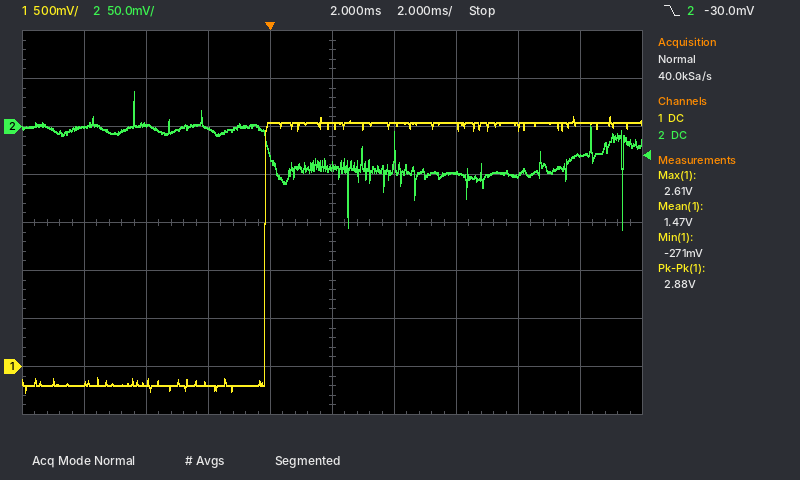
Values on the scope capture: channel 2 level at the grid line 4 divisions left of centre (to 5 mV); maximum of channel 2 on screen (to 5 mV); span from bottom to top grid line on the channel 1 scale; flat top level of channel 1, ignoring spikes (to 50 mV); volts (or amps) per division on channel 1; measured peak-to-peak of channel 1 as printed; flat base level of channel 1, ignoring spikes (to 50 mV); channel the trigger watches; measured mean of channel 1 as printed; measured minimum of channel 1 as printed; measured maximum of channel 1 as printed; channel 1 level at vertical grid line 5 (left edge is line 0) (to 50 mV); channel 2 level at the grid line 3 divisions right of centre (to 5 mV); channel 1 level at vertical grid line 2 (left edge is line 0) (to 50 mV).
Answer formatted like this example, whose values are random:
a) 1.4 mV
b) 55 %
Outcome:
a) 0 mV
b) 35 mV
c) 4 V
d) 2.55 V
e) 500 mV
f) 2.88 V
g) -200 mV
h) channel 2
i) 1.47 V
j) -271 mV
k) 2.61 V
l) 2.50 V
m) -50 mV
n) -150 mV
